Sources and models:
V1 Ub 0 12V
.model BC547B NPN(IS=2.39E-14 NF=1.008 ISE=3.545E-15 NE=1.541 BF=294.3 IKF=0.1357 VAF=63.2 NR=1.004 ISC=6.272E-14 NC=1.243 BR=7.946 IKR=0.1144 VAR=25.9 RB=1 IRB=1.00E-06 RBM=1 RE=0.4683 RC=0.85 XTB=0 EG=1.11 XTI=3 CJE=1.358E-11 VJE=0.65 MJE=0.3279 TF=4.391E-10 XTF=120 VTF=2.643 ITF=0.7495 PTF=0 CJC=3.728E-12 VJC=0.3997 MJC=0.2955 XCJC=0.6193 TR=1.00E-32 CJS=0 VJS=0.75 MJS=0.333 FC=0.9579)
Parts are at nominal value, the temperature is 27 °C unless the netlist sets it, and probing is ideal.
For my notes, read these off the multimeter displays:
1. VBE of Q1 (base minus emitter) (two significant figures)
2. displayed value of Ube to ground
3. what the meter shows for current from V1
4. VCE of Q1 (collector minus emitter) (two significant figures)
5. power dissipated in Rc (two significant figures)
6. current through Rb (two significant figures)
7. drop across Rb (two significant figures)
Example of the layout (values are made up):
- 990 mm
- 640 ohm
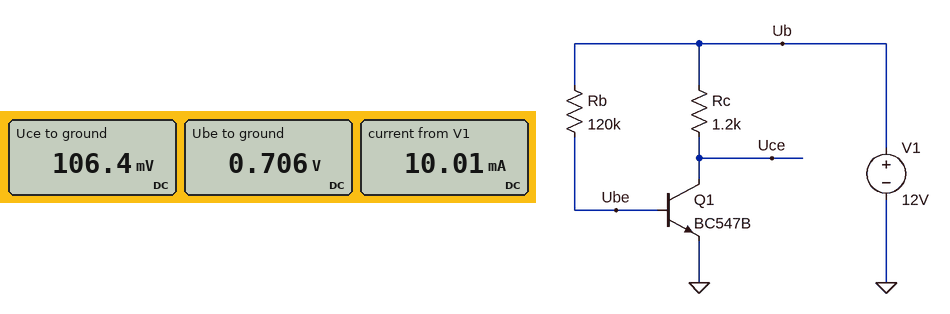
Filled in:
- 710 mV
- 0.706 V
- 10.01 mA
- 110 mV
- 120 mW
- 94 µA
- 11 V
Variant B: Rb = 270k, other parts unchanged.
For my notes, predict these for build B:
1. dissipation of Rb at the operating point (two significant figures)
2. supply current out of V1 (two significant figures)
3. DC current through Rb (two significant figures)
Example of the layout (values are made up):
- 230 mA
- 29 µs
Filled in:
- 470 µW
- 9.9 mA
- 42 µA
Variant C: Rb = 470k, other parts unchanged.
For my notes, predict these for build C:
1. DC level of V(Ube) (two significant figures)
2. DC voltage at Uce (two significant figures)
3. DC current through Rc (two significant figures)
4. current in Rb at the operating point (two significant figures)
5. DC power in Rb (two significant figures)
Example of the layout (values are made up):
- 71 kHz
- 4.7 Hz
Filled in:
- 690 mV
- 3.8 V
- 6.9 mA
- 24 µA
- 270 µW
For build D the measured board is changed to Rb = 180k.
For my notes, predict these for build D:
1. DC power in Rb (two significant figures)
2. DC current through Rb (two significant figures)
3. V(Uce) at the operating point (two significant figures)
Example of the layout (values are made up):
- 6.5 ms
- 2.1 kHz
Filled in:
- 710 µW
- 63 µA
- 130 mV
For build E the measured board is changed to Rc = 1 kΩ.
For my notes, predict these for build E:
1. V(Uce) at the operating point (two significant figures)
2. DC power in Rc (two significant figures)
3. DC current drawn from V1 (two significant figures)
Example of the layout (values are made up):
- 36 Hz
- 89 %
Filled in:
- 120 mV
- 140 mW
- 12 mA
